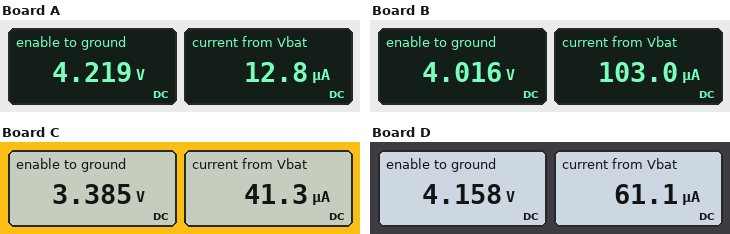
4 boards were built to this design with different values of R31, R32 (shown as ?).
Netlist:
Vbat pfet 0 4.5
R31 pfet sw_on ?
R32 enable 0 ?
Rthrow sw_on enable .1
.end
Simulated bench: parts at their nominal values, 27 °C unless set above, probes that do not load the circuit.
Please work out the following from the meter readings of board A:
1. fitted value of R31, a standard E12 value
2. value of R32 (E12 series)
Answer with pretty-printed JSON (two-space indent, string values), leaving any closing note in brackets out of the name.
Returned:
{
  "fitted value of R31, a standard E12 value": "22 kΩ",
  "value of R32": "330 kΩ"
}
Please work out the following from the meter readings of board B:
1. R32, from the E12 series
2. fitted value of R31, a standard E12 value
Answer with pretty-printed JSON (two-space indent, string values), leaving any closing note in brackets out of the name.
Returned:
{
  "R32, from the E12 series": "39 kΩ",
  "fitted value of R31, a standard E12 value": "4.7 kΩ"
}
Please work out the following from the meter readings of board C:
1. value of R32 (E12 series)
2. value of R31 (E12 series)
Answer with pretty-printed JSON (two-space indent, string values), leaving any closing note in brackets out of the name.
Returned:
{
  "value of R32": "82 kΩ",
  "value of R31": "27 kΩ"
}
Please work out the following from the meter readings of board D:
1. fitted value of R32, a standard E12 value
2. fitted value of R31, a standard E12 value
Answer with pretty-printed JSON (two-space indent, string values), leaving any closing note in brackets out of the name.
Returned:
{
  "fitted value of R32, a standard E12 value": "68 kΩ",
  "fitted value of R31, a standard E12 value": "5.6 kΩ"
}
